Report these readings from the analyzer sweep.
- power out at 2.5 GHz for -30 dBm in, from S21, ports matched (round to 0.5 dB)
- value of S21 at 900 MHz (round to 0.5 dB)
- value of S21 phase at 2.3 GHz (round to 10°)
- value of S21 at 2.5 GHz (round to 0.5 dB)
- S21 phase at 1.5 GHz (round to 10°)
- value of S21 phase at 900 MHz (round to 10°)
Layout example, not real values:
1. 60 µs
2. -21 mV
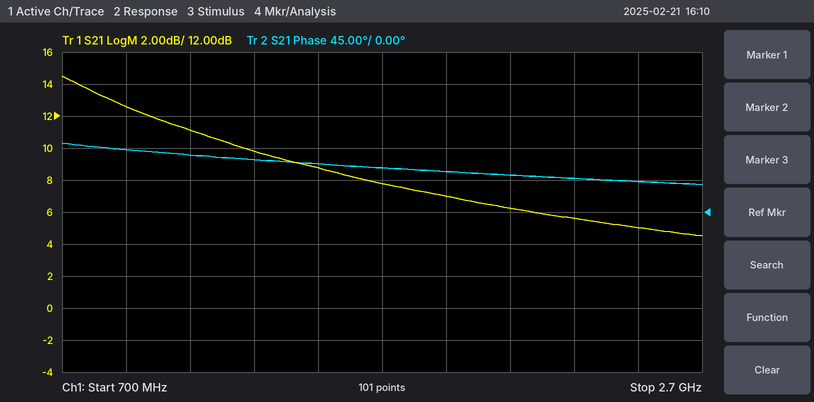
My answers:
1. -25.0 dBm
2. 12.5 dB
3. 50°
4. 5.0 dB
5. 70°
6. 90°
